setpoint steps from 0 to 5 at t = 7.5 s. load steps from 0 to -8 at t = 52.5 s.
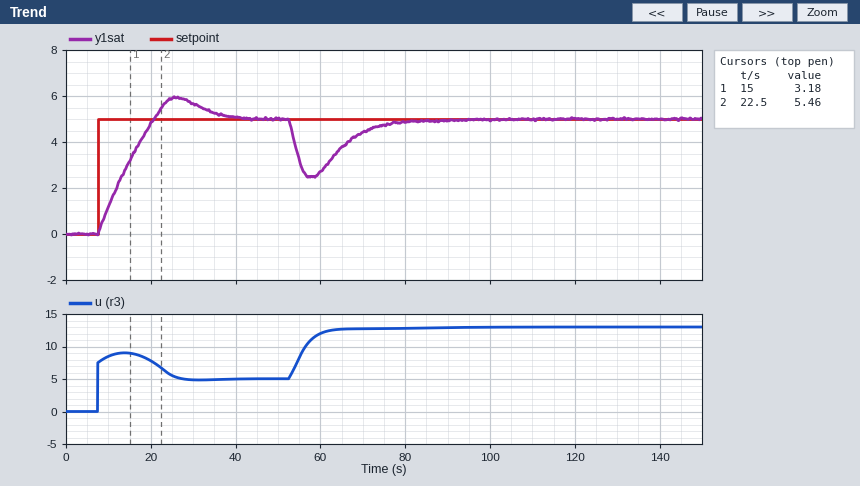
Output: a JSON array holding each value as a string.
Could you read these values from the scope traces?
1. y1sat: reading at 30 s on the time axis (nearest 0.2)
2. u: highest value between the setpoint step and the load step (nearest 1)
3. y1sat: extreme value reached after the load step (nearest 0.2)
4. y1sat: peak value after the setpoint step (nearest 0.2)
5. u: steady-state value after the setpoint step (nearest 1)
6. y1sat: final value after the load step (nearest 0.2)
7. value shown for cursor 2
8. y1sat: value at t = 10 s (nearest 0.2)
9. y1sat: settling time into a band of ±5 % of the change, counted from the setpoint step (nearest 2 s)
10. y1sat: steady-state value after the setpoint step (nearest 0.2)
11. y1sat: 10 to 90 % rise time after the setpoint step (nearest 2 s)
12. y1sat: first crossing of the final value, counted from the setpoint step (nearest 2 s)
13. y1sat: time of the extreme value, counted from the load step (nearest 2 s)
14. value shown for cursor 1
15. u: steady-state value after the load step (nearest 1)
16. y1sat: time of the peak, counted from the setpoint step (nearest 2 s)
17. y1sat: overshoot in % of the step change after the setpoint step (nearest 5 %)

["5.6", "9", "2.4", "6.0", "5", "5.0", "5.46", "1.2", "28 s", "5.0", "10 s", "14 s", "6 s", "3.18", "13", "18 s", "20 %"]
